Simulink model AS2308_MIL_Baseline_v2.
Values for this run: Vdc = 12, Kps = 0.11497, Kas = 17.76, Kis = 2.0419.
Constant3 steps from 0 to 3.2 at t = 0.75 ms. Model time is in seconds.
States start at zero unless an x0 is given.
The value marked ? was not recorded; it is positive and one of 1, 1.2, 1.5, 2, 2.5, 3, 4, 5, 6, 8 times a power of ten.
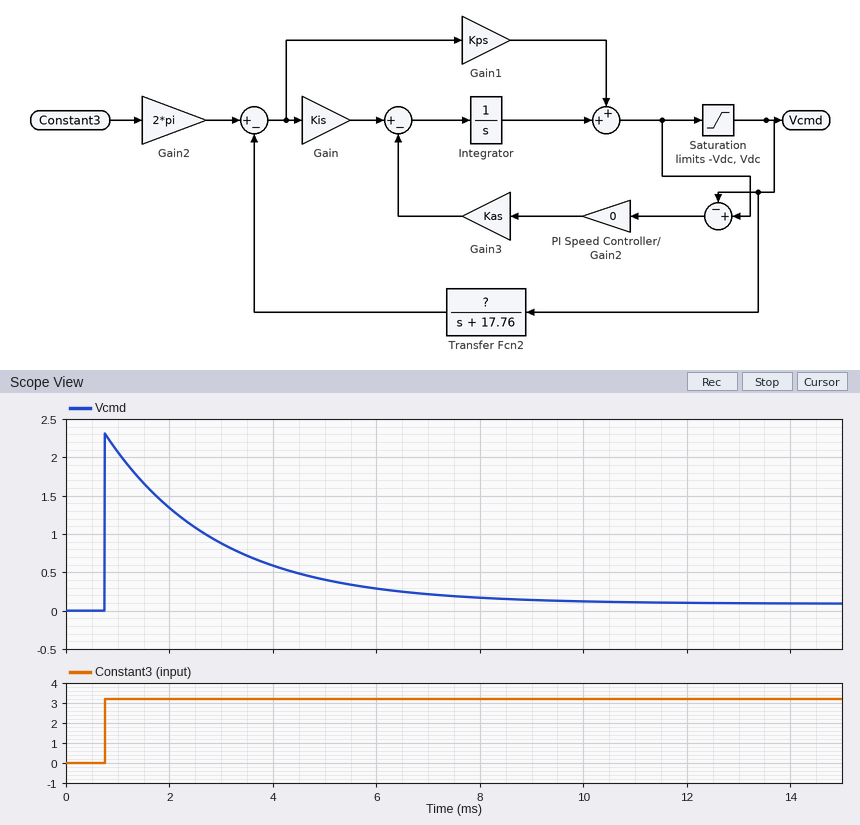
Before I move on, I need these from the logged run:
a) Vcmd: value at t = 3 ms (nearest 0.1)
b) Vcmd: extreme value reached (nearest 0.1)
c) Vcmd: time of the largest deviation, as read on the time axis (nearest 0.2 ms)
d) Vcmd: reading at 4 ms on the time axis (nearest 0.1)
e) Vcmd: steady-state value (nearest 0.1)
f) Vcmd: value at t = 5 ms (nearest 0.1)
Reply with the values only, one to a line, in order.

0.9
2.3
0.8 ms
0.6
0.1
0.4
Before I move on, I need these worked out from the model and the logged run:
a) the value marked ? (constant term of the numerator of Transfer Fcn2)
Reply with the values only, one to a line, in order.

4000
